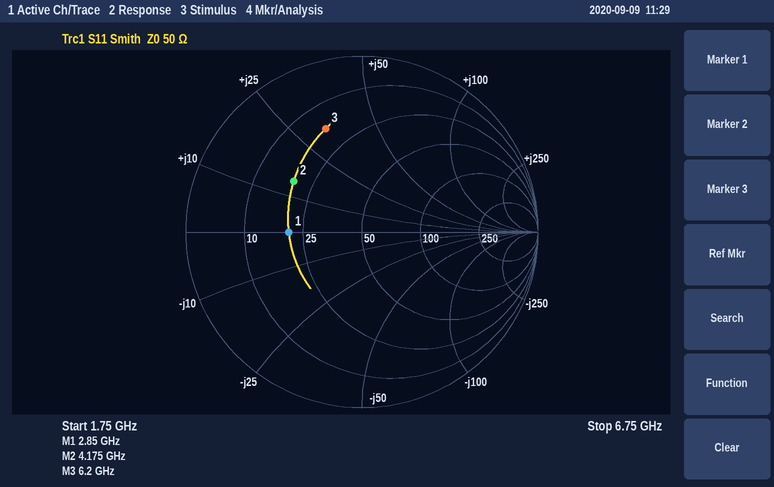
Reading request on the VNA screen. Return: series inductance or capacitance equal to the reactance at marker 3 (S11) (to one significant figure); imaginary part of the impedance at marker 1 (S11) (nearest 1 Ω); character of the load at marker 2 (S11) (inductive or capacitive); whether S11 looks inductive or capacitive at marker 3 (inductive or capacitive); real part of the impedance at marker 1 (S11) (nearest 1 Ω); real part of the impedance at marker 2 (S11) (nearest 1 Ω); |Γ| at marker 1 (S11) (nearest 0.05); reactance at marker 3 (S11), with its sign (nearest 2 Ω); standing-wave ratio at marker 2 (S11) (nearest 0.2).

800 pH
0 Ω
inductive
inductive
21 Ω
19 Ω
0.40
+32 Ω
2.8
